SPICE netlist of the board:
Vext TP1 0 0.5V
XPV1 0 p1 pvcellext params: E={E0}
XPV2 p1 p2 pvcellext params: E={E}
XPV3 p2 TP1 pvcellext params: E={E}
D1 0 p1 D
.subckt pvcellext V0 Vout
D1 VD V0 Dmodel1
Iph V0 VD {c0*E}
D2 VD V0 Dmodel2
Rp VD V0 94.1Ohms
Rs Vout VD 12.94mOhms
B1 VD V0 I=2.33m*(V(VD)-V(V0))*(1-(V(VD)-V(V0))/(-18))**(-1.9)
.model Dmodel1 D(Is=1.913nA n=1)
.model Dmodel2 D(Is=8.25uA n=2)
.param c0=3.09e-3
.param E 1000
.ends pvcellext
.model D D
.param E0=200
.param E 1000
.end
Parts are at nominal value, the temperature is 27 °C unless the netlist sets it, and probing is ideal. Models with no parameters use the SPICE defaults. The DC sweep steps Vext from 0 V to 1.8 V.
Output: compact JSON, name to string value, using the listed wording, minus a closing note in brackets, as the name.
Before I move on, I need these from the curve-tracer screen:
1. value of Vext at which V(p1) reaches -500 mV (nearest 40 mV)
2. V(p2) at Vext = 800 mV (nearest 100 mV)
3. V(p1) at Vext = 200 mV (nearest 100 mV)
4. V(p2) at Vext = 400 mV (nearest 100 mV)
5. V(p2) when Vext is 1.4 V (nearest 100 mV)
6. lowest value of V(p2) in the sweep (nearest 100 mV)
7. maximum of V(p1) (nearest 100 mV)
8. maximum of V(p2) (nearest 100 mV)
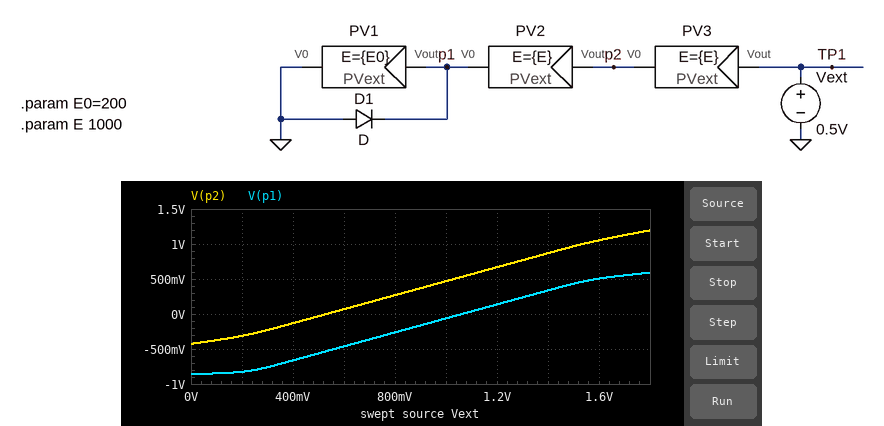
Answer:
{"value of Vext at which V(p1) reaches -500 mV": "560 mV", "V(p2) at Vext = 800 mV": "300 mV", "V(p1) at Vext = 200 mV": "-800 mV", "V(p2) at Vext = 400 mV": "-100 mV", "V(p2) when Vext is 1.4 V": "900 mV", "lowest value of V(p2) in the sweep": "-400 mV", "maximum of V(p1)": "600 mV", "maximum of V(p2)": "1.2 V"}
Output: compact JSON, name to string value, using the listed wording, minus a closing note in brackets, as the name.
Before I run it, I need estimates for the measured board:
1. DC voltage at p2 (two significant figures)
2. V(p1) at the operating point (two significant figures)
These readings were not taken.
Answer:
{"DC voltage at p2": "-31 mV", "V(p1) at the operating point": "-560 mV"}
